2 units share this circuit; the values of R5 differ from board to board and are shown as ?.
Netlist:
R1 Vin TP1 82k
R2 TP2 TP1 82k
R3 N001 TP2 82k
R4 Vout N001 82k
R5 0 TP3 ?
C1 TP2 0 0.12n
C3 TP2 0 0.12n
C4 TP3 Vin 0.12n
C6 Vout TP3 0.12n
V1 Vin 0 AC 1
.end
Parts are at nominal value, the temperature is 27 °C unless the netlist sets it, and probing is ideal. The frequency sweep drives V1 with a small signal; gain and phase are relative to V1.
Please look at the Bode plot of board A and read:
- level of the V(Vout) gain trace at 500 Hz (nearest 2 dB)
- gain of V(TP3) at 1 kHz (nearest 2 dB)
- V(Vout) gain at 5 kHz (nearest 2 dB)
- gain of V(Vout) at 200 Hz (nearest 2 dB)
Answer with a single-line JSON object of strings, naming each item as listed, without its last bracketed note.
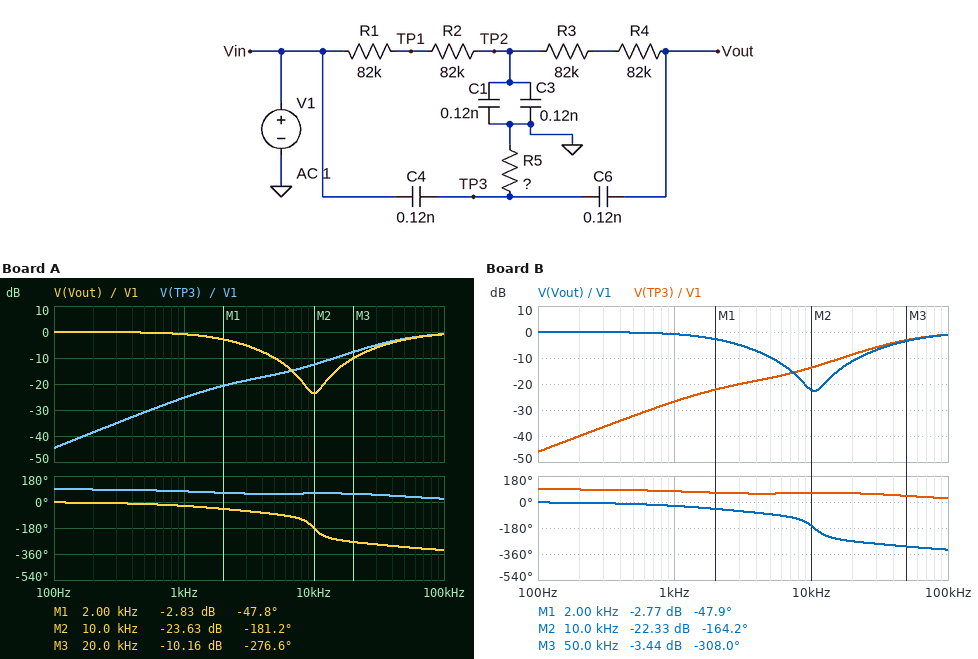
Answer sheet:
{"level of the V(Vout) gain trace at 500 Hz": "0 dB", "gain of V(TP3) at 1 kHz": "-26 dB", "V(Vout) gain at 5 kHz": "-10 dB", "gain of V(Vout) at 200 Hz": "0 dB"}
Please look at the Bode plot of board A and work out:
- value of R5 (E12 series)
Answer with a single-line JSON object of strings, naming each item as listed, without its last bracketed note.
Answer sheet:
{"value of R5": "39 kΩ"}
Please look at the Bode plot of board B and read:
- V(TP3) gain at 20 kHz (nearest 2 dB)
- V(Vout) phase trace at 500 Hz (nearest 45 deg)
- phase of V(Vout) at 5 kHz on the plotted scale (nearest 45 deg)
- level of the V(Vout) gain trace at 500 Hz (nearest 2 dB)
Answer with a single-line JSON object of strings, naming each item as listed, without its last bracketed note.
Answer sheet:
{"V(TP3) gain at 20 kHz": "-8 dB", "V(Vout) phase trace at 500 Hz": "0 deg", "phase of V(Vout) at 5 kHz on the plotted scale": "-90 deg", "level of the V(Vout) gain trace at 500 Hz": "0 dB"}
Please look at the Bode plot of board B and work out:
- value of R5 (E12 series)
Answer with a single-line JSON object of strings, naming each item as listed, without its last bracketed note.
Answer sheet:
{"value of R5": "33 kΩ"}
